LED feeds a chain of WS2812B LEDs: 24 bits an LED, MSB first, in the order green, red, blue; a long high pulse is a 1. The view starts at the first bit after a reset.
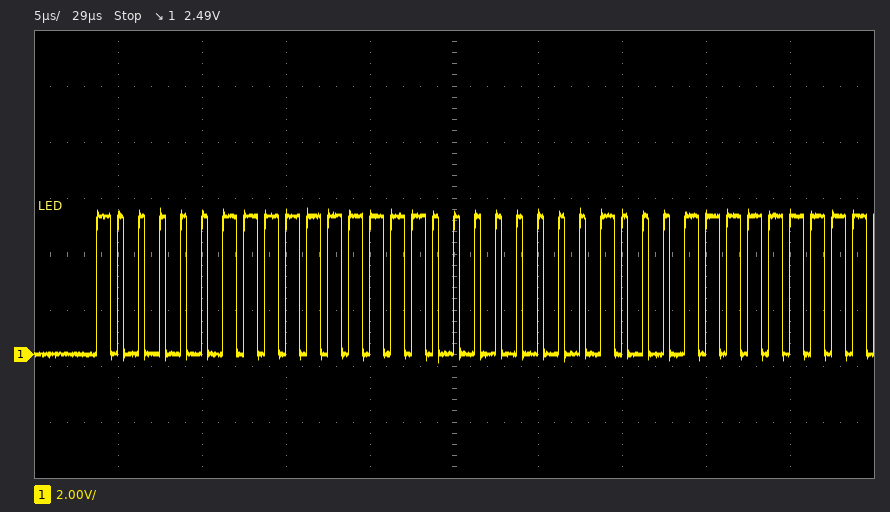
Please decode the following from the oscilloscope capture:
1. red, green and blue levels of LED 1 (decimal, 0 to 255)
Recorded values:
255, 131, 0
